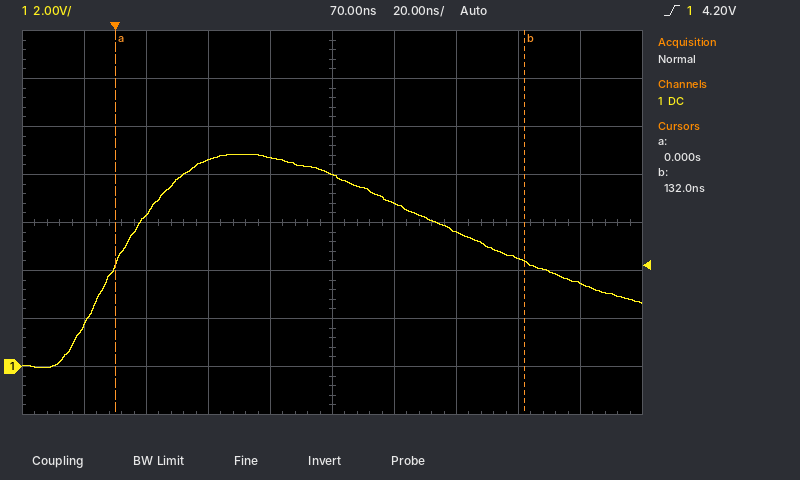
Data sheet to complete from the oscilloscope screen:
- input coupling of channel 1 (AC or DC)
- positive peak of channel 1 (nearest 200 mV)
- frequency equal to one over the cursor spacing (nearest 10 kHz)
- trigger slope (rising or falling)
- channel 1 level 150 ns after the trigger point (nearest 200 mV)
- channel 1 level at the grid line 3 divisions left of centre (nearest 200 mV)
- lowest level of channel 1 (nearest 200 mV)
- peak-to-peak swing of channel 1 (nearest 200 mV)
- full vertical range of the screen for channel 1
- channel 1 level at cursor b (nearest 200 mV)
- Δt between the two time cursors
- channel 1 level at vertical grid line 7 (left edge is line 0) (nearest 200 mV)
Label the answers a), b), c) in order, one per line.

a) DC
b) 8.8 V
c) 7.58 MHz
d) rising
e) 3.4 V
f) 6.4 V
g) 0.0 V
h) 8.8 V
i) 16 V
j) 4.4 V
k) 132 ns
l) 5.6 V
